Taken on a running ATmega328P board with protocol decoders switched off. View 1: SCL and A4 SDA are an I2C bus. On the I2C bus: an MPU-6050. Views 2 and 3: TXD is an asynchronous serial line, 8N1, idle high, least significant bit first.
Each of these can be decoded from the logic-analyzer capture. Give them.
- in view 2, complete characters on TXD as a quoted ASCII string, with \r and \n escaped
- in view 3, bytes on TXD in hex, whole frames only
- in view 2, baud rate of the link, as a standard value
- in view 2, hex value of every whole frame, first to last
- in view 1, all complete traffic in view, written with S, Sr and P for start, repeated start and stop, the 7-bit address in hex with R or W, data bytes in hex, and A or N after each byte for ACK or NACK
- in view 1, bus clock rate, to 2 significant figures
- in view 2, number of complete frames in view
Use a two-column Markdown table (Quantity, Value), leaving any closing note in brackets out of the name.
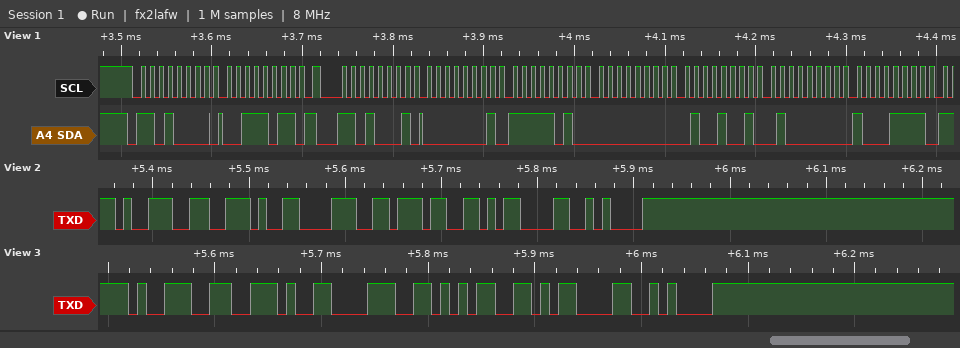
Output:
| Quantity | Value |
|---|---|
| in view 2, complete characters on TXD as a quoted ASCII string, with \r and \n escaped | "9.87\r\n" |
| in view 3, bytes on TXD in hex, whole frames only | 0x39 0x2E 0x38 0x35 0x0D 0x0A |
| in view 2, baud rate of the link, as a standard value | 115200 baud |
| in view 2, hex value of every whole frame, first to last | 39 2E 38 37 0D 0A |
| in view 1, all complete traffic in view, written with S, Sr and P for start, repeated start and stop, the 7-bit address in hex with R or W, data bytes in hex, and A or N after each byte for ACK or NACK | S 68W A 3B A Sr 68R A 01 A FA A 00 A 49 A 40 A 8F A |
| in view 1, bus clock rate, to 2 significant figures | 100 kHz |
| in view 2, number of complete frames in view | 6 |
